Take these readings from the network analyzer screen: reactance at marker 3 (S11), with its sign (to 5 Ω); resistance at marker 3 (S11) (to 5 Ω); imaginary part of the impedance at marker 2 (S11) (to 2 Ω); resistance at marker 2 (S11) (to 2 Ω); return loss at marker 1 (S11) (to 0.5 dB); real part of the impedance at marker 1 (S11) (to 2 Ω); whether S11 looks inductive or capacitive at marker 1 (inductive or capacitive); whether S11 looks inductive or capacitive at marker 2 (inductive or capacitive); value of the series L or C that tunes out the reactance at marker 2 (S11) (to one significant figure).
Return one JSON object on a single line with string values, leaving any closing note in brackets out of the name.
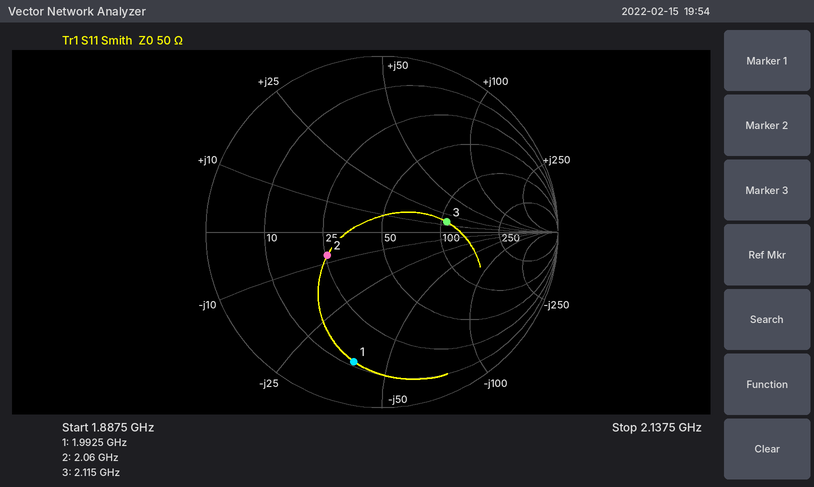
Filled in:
{"reactance at marker 3 (S11), with its sign": "+15 Ω", "resistance at marker 3 (S11)": "105 Ω", "imaginary part of the impedance at marker 2 (S11)": "-8 Ω", "resistance at marker 2 (S11)": "26 Ω", "return loss at marker 1 (S11)": "2.5 dB", "real part of the impedance at marker 1 (S11)": "12 Ω", "whether S11 looks inductive or capacitive at marker 1": "capacitive", "whether S11 looks inductive or capacitive at marker 2": "capacitive", "value of the series L or C that tunes out the reactance at marker 2 (S11)": "600 pH"}
